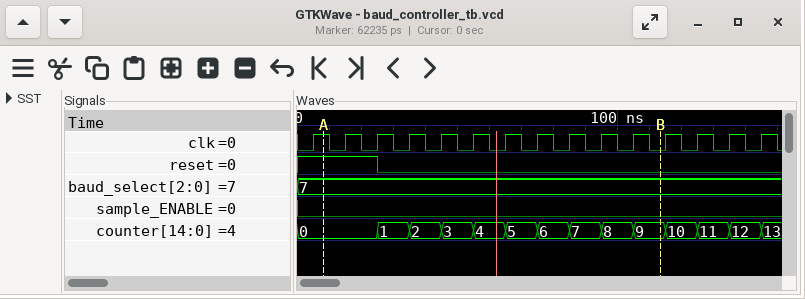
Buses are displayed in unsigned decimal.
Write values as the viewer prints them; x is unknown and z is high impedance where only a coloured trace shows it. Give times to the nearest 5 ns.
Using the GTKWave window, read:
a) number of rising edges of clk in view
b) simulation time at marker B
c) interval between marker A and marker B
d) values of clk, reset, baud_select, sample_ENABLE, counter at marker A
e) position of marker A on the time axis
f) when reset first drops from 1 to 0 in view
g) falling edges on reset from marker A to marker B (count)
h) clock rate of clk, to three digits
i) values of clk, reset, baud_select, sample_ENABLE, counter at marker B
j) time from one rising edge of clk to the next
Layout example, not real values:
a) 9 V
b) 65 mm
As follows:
a) 15
b) 115 ns
c) 105 ns
d) clk=1, reset=1, baud_select=7, sample_ENABLE=0, counter=0
e) 10 ns
f) 25 ns
g) 1
h) 100 MHz
i) clk=0, reset=0, baud_select=7, sample_ENABLE=0, counter=9
j) 10 ns
